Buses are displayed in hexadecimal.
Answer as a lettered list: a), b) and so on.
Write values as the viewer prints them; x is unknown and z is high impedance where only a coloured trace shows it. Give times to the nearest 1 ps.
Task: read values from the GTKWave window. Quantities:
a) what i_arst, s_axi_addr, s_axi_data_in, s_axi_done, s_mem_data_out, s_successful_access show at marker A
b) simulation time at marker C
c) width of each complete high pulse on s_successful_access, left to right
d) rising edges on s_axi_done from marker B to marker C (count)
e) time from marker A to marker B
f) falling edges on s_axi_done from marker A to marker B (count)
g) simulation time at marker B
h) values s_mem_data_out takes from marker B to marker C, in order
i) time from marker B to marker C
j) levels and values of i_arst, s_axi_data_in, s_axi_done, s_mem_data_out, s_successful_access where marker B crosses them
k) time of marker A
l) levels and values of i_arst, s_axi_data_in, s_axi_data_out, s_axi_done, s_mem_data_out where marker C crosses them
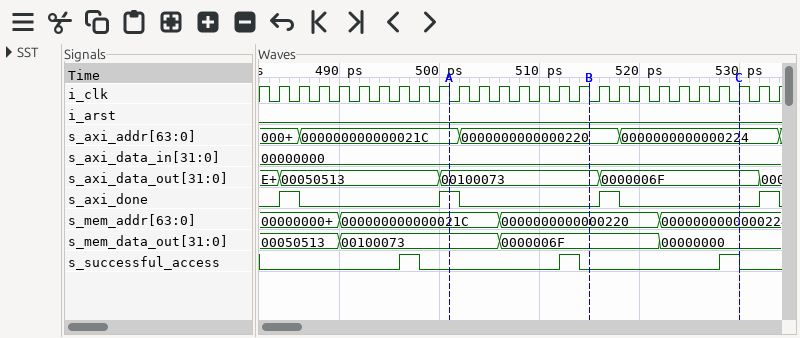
a) i_arst=0, s_axi_addr=000000000000021C, s_axi_data_in=00000000, s_axi_done=1, s_mem_data_out=00100073, s_successful_access=0
b) 530 ps
c) 2 ps, 2 ps, 2 ps
d) 1
e) 14 ps
f) 1
g) 515 ps
h) 0000006F, 00000000
i) 15 ps
j) i_arst=0, s_axi_data_in=00000000, s_axi_done=0, s_mem_data_out=0000006F, s_successful_access=0
k) 501 ps
l) i_arst=0, s_axi_data_in=00000000, s_axi_data_out=0000006F, s_axi_done=0, s_mem_data_out=00000000
